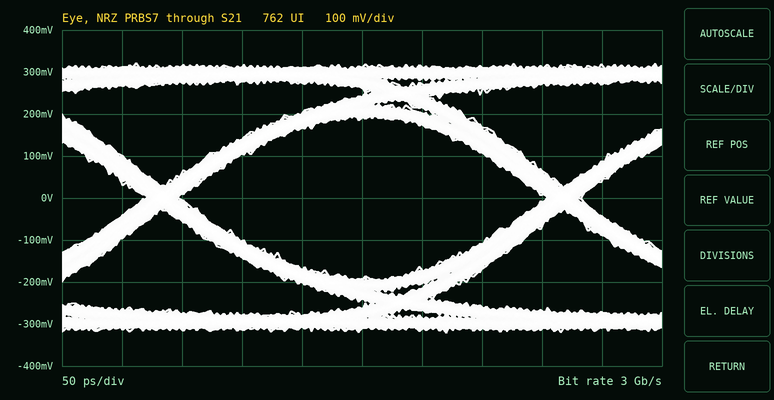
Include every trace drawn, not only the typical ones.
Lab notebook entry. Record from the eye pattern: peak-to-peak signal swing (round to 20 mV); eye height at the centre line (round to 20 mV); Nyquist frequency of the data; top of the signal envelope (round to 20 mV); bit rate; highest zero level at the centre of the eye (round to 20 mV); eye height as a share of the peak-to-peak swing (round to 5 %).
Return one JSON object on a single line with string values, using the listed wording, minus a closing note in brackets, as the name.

{"peak-to-peak signal swing": "640 mV", "eye height at the centre line": "380 mV", "Nyquist frequency of the data": "1.5 GHz", "top of the signal envelope": "320 mV", "bit rate": "3 Gb/s", "highest zero level at the centre of the eye": "-200 mV", "eye height as a share of the peak-to-peak swing": "60 %"}
